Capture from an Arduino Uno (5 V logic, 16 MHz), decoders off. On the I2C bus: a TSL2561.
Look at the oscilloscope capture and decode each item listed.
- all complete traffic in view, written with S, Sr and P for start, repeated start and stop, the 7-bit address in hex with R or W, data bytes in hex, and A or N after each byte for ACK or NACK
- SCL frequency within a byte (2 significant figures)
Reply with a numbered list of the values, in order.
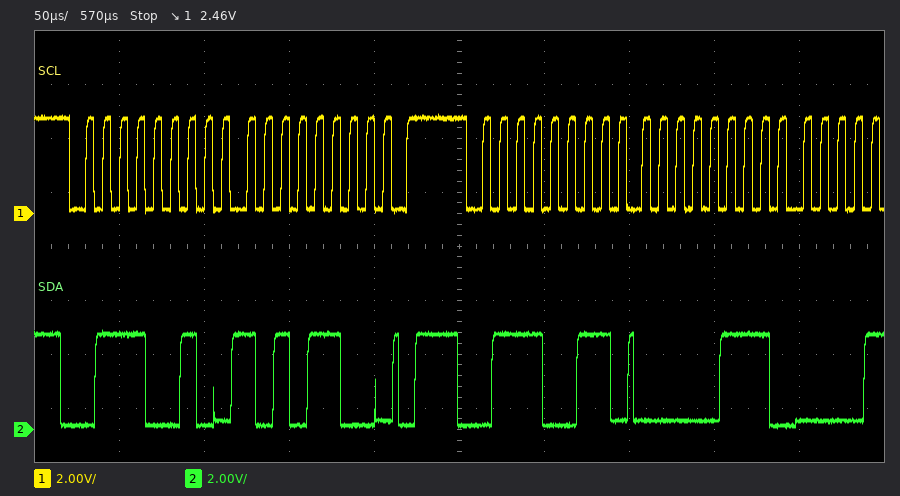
1. S 39W A AC A P S 39R A 07 A
2. 100 kHz
